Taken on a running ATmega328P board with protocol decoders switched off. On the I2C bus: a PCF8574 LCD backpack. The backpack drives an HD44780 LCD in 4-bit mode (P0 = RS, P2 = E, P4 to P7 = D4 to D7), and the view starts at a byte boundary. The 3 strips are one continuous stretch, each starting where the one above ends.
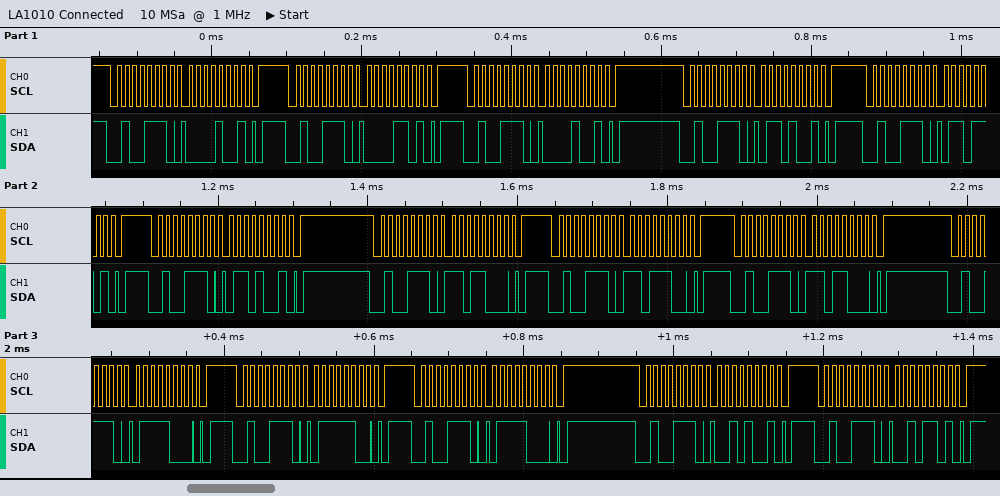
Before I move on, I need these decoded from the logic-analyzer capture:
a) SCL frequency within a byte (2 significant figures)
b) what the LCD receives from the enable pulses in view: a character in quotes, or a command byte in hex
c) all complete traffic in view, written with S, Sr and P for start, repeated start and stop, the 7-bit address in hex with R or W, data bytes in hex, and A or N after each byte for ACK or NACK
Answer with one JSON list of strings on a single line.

["100 kHz", "data 0x06 0xD7", "S 27W A 09 A P S 27W A 0D A P S 27W A 09 A P S 27W A 69 A P S 27W A 6D A P S 27W A 69 A P S 27W A D8 A P S 27W A DC A P S 27W A D8 A P S 27W A 78 A P S 27W A 7C A P S 27W A 78 A P S 27W A 29 A P S 27W A 2D A P"]
